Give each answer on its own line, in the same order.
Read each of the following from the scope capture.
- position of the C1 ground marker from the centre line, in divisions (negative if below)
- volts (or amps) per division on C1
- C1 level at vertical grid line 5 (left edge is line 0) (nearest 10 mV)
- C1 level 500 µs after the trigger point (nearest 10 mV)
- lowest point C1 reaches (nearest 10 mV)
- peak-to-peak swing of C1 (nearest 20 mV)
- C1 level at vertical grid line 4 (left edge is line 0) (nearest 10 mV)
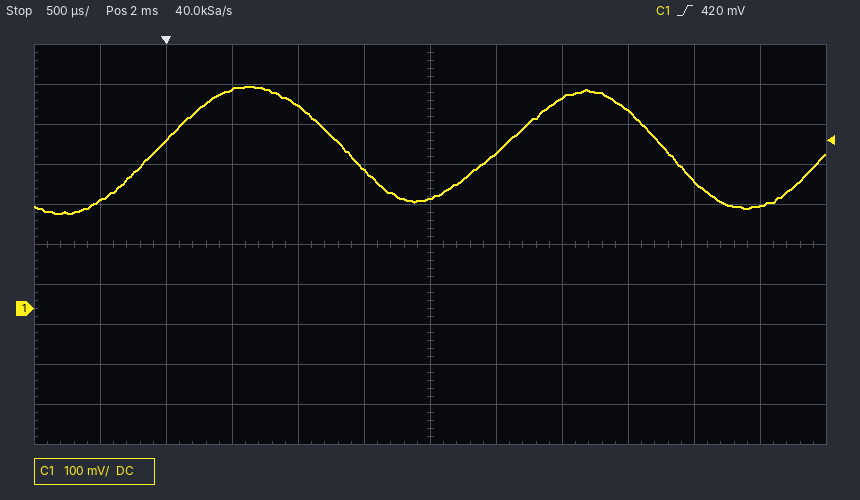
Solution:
-1.6 div
100 mV
350 mV
550 mV
240 mV
320 mV
510 mV
